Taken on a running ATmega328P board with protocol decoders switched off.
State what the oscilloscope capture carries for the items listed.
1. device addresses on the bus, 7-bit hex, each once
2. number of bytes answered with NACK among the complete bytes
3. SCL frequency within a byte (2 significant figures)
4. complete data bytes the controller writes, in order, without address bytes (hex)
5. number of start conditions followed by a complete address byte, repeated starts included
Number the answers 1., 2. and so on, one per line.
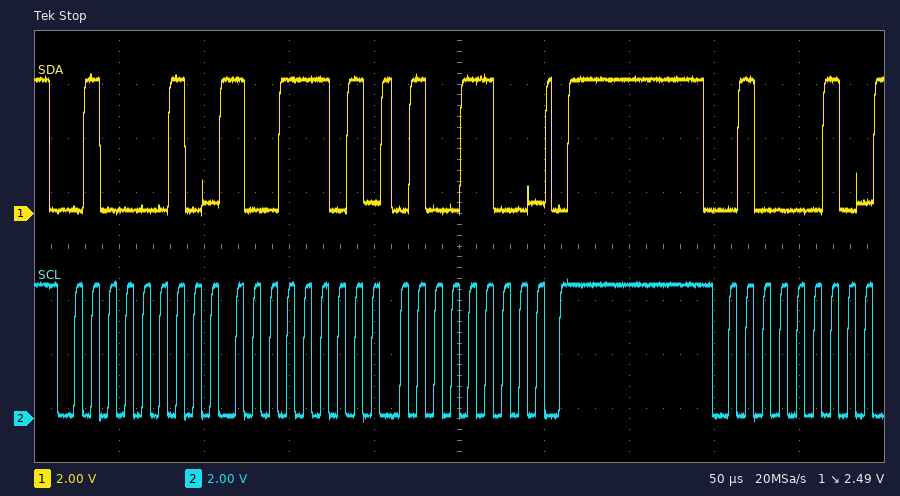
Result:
1. 0x21
2. 0
3. 100 kHz
4. 9D 4C
5. 2
